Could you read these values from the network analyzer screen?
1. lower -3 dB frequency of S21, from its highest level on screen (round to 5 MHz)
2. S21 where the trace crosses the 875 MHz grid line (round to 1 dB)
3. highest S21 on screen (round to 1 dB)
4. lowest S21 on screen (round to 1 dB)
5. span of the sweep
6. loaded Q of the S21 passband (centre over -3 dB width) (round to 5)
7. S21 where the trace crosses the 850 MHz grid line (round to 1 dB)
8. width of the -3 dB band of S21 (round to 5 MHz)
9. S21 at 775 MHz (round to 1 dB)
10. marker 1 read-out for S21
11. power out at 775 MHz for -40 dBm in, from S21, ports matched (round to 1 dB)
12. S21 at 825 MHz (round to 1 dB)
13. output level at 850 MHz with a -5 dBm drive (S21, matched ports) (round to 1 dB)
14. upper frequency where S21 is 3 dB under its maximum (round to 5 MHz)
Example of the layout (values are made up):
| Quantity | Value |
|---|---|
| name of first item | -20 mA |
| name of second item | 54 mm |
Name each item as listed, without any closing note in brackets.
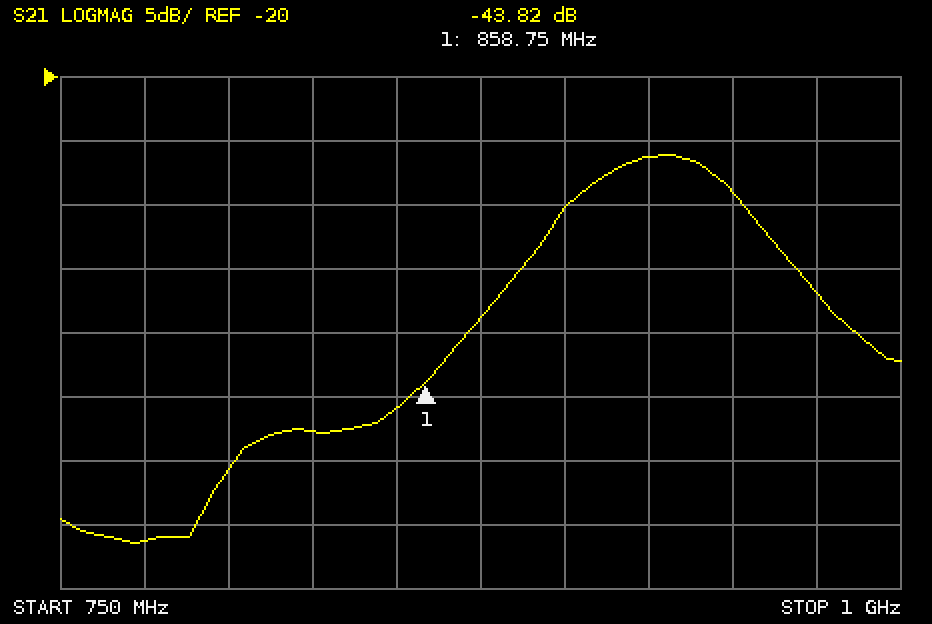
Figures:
| Quantity | Value |
|---|---|
| lower -3 dB frequency of S21, from its highest level on screen | 905 MHz |
| S21 where the trace crosses the 875 MHz grid line | -39 dB |
| highest S21 on screen | -26 dB |
| lowest S21 on screen | -56 dB |
| span of the sweep | 250 MHz |
| loaded Q of the S21 passband (centre over -3 dB width) | 20 |
| S21 where the trace crosses the 850 MHz grid line | -46 dB |
| width of the -3 dB band of S21 | 45 MHz |
| S21 at 775 MHz | -56 dB |
| marker 1 read-out for S21 | -43.82 dB |
| power out at 775 MHz for -40 dBm in, from S21, ports matched | -96 dBm |
| S21 at 825 MHz | -48 dB |
| output level at 850 MHz with a -5 dBm drive (S21, matched ports) | -51 dBm |
| upper frequency where S21 is 3 dB under its maximum | 950 MHz |
